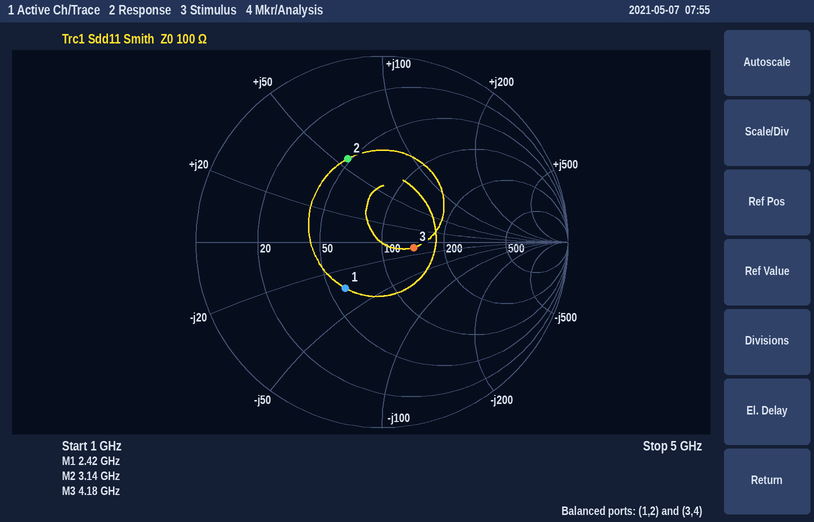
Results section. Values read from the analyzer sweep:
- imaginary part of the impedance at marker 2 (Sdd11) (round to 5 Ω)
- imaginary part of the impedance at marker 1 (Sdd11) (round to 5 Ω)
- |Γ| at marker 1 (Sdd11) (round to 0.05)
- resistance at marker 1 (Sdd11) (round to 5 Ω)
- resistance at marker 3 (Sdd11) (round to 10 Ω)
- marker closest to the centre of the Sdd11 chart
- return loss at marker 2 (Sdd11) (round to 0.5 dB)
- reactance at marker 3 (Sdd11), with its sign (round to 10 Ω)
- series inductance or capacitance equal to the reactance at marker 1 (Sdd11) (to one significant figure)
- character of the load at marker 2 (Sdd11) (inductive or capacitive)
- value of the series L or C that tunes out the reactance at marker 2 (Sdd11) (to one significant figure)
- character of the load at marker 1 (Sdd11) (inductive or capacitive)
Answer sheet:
+55 Ω
-35 Ω
0.30
60 Ω
140 Ω
marker 3
6.5 dB
-10 Ω
2 pF
inductive
900 fF
capacitive
